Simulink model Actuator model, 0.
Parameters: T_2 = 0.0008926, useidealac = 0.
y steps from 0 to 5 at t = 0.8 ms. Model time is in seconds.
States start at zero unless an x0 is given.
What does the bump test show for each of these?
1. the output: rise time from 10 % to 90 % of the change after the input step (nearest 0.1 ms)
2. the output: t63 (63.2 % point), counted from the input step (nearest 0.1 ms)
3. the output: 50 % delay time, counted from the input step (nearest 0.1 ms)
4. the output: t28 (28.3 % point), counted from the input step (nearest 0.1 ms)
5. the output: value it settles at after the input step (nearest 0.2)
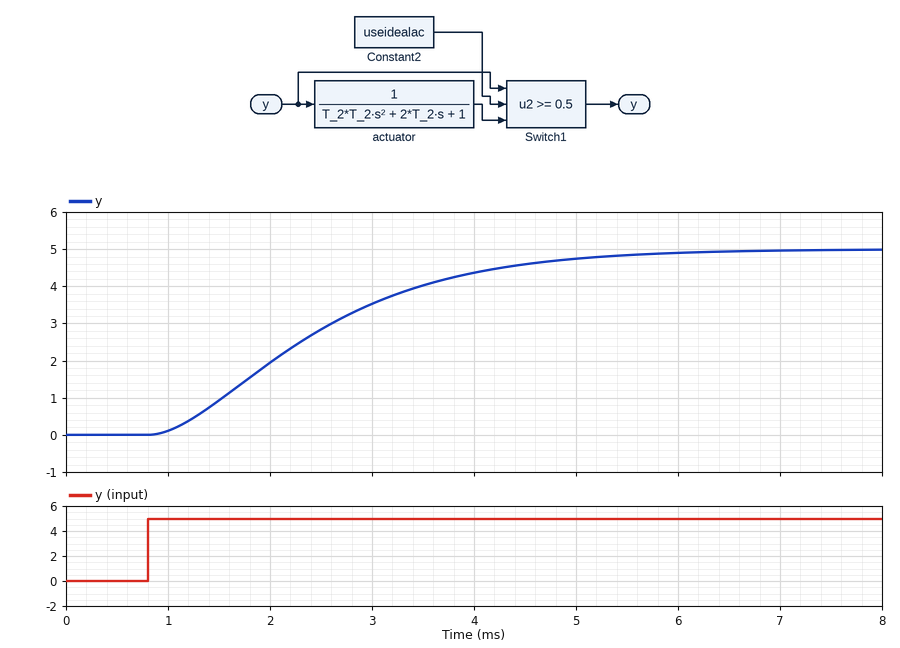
3.0 ms
1.9 ms
1.5 ms
0.9 ms
5.0
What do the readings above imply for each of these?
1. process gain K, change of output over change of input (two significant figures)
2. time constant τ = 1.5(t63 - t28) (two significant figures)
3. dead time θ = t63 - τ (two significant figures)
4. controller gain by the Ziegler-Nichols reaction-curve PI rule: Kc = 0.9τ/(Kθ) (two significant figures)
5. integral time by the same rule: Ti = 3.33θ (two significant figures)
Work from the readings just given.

1.0
1.5 ms
0.40 ms
3.4
1.3 ms
